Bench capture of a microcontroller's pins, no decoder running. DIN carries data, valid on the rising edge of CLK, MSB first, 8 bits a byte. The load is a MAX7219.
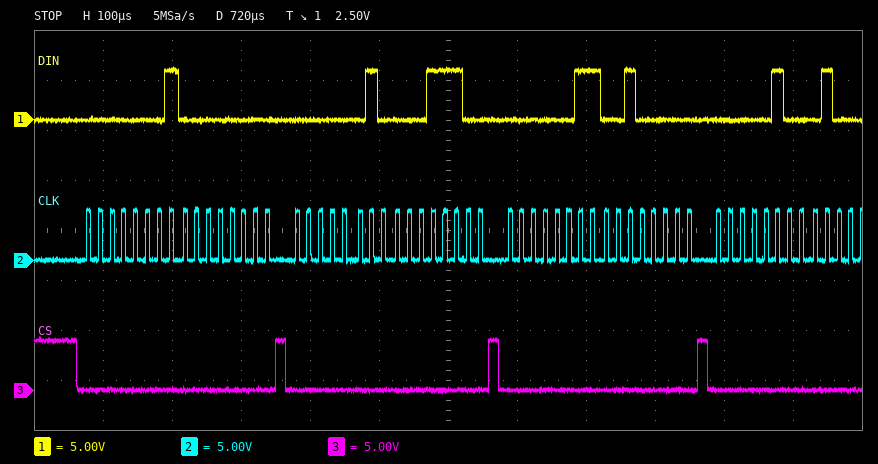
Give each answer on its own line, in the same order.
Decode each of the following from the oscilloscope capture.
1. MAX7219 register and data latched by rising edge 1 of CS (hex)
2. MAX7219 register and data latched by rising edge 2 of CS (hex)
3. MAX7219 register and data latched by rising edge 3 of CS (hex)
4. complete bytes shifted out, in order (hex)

register 0x1, data 0x00
register 0x2, data 0x1C
register 0x3, data 0x20
0x01 0x00 0x02 0x1C 0x03 0x20 0x04
